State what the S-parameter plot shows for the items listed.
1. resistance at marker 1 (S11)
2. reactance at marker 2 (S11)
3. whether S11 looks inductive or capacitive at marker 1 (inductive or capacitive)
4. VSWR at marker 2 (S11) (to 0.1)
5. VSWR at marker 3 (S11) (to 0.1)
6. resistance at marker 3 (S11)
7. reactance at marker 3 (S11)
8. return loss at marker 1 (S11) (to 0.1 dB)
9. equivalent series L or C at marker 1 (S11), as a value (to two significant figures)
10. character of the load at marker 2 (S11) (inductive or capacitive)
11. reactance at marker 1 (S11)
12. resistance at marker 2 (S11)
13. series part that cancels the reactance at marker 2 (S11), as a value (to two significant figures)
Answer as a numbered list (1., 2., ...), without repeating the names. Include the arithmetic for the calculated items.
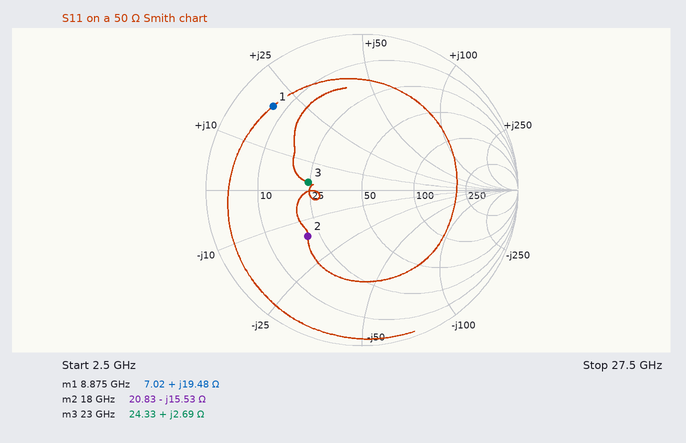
1. 7.02 Ω
2. -15.53 Ω
3. inductive
4. 2.7
5. 2.1
6. 24.33 Ω
7. +2.69 Ω
8. 2.1 dB
9. L = 19.48 Ω/(2π × 8.875 GHz) ≈ 349 pH, so 350 pH to two significant figures
10. capacitive
11. +19.48 Ω
12. 20.83 Ω
13. L = 15.53 Ω/(2π × 18 GHz) ≈ 137 pH, so 140 pH to two significant figures
